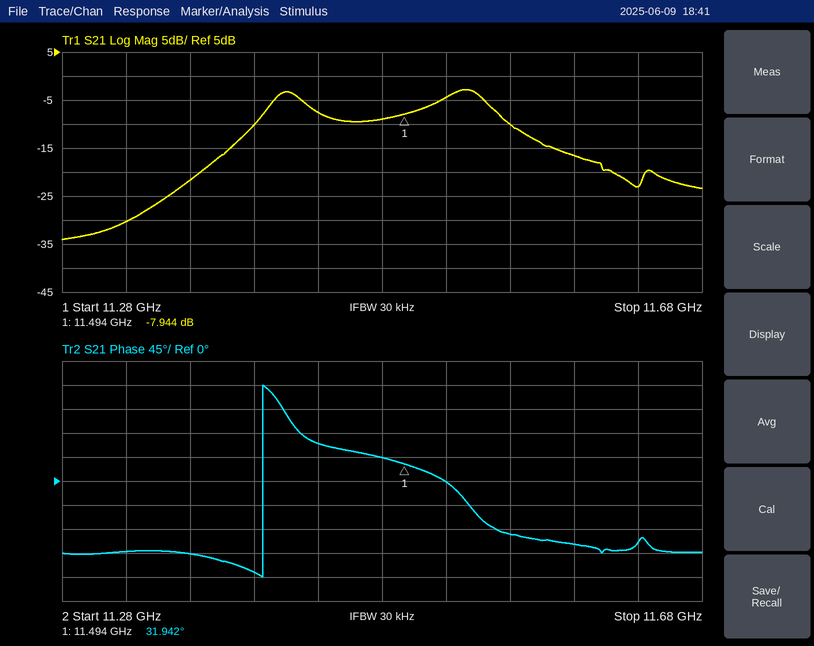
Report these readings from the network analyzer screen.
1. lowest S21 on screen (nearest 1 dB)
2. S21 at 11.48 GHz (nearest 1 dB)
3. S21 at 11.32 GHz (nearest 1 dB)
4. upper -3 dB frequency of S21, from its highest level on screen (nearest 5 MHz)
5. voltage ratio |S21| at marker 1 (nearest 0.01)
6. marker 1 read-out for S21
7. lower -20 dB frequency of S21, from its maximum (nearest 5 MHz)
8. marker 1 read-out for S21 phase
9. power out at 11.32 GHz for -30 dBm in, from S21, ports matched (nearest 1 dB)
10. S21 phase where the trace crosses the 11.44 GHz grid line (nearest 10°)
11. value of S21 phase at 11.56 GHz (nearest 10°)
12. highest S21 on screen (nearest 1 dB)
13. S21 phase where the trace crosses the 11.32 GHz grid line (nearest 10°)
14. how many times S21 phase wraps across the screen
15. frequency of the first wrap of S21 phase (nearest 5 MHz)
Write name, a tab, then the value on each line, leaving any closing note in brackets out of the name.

lowest S21 on screen	-34 dB
S21 at 11.48 GHz	-9 dB
S21 at 11.32 GHz	-30 dB
upper -3 dB frequency of S21, from its highest level on screen	11.545 GHz
voltage ratio |S21| at marker 1	0.40
marker 1 read-out for S21	-7.944 dB
lower -20 dB frequency of S21, from its maximum	11.355 GHz
marker 1 read-out for S21 phase	31.942°
power out at 11.32 GHz for -30 dBm in, from S21, ports matched	-60 dBm
S21 phase where the trace crosses the 11.44 GHz grid line	70°
value of S21 phase at 11.56 GHz	-100°
highest S21 on screen	-3 dB
S21 phase where the trace crosses the 11.32 GHz grid line	-130°
how many times S21 phase wraps across the screen	1
frequency of the first wrap of S21 phase	11.405 GHz
